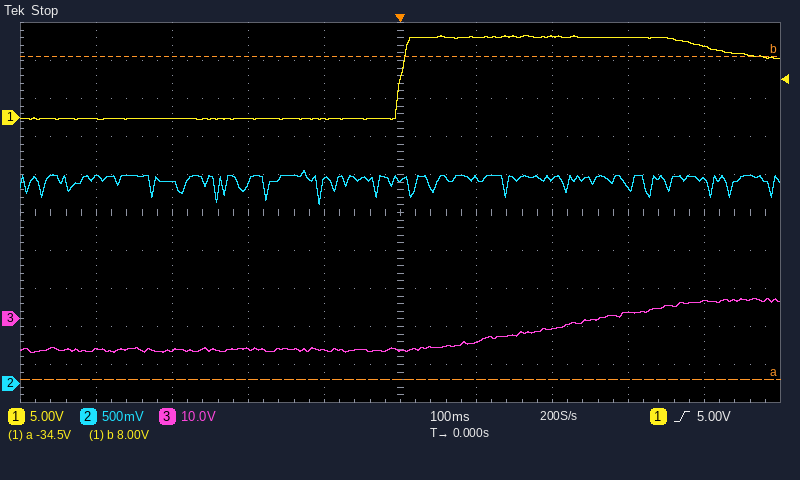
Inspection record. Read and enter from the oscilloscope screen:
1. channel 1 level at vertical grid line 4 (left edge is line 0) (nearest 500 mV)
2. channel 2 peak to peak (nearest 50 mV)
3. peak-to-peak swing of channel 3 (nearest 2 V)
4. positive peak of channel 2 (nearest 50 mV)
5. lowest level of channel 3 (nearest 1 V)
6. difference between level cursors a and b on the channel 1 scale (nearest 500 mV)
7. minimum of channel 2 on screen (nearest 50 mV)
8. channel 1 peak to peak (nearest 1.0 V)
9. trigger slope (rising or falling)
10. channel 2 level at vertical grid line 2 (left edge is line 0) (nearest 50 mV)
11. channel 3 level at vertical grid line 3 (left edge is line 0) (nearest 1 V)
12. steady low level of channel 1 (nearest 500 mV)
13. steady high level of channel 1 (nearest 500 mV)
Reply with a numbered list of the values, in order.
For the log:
1. 0.0 V
2. 450 mV
3. 14 V
4. 2.80 V
5. -9 V
6. 42.5 V
7. 2.35 V
8. 11.0 V
9. rising
10. 2.65 V
11. -8 V
12. 0.0 V
13. 10.5 V
